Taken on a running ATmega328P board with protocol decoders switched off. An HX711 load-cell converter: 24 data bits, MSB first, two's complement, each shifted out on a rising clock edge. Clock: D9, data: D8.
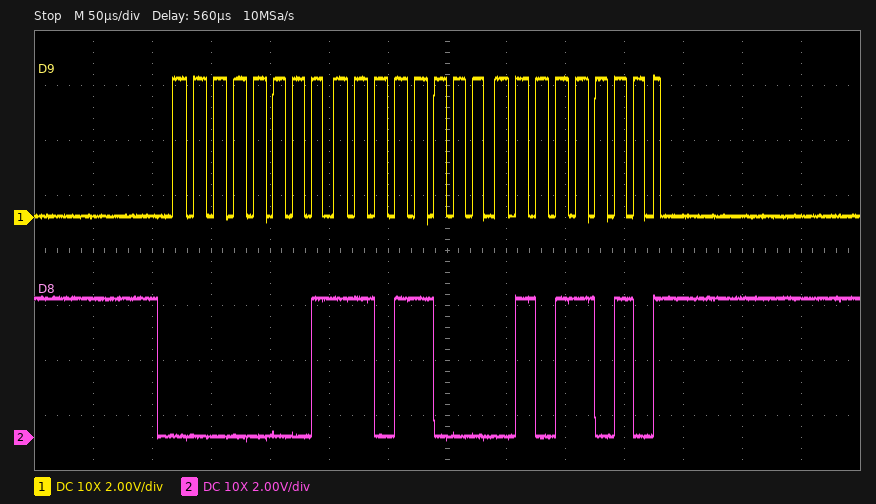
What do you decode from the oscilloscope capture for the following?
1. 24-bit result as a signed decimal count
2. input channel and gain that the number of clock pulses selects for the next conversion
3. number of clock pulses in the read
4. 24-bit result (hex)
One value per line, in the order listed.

120922
channel A, gain 128
25
0x01D85A
